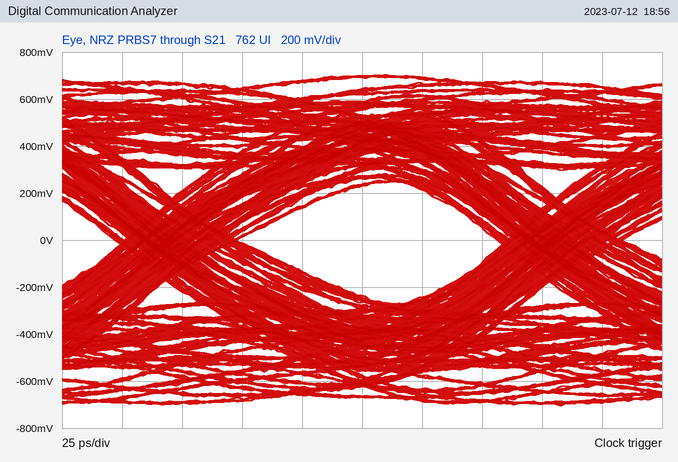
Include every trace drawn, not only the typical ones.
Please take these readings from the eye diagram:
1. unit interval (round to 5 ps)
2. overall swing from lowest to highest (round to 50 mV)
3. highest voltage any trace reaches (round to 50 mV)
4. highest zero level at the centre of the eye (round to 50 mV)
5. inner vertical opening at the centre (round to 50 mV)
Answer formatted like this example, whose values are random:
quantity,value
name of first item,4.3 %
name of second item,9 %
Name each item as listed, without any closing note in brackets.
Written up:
quantity,value
unit interval,160 ps
overall swing from lowest to highest,1.40 V
highest voltage any trace reaches,700 mV
highest zero level at the centre of the eye,-250 mV
inner vertical opening at the centre,450 mV
